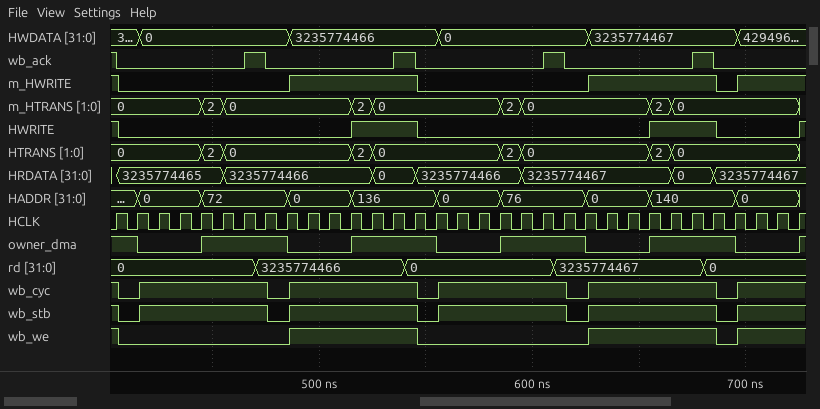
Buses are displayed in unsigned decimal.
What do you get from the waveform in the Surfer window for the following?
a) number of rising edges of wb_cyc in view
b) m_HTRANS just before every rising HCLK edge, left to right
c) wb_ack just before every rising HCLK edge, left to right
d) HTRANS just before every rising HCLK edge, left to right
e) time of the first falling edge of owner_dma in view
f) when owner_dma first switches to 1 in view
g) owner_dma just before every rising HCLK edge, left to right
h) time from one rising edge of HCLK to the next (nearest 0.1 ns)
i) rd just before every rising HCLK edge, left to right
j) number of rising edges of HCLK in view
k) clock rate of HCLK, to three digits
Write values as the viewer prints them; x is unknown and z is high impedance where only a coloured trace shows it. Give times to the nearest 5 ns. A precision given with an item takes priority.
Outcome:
5
0, 0, 0, 0, 0, 2, 0, 0, 0, 0, 0, 0, 2, 0, 0, 0, 0, 0, 0, 2, 0, 0, 0, 0, 0, 0, 2, 0, 0, 0, 0, 0, 0
1 0 0 0 0 0 0 1 0 0 0 0 0 0 1 0 0 0 0 0 0 1 0 0 0 0 0 0 1 0 0 0 0
0, 0, 0, 0, 0, 2, 0, 0, 0, 0, 0, 0, 2, 0, 0, 0, 0, 0, 0, 2, 0, 0, 0, 0, 0, 0, 2, 0, 0, 0, 0, 0, 0
415 ns
445 ns
1 1 0 0 0 1 1 1 1 0 0 0 1 1 1 1 0 0 0 1 1 1 1 0 0 0 1 1 1 1 0 0 0
10 ns
0, 0, 0, 0, 0, 0, 0, 3235774466, 3235774466, 3235774466, 3235774466, 3235774466, 3235774466, 3235774466, 0, 0, 0, 0, 0, 0, 0, 3235774467, 3235774467, 3235774467, 3235774467, 3235774467, 3235774467, 3235774467, 0, 0, 0, 0, 0
33
100 MHz
